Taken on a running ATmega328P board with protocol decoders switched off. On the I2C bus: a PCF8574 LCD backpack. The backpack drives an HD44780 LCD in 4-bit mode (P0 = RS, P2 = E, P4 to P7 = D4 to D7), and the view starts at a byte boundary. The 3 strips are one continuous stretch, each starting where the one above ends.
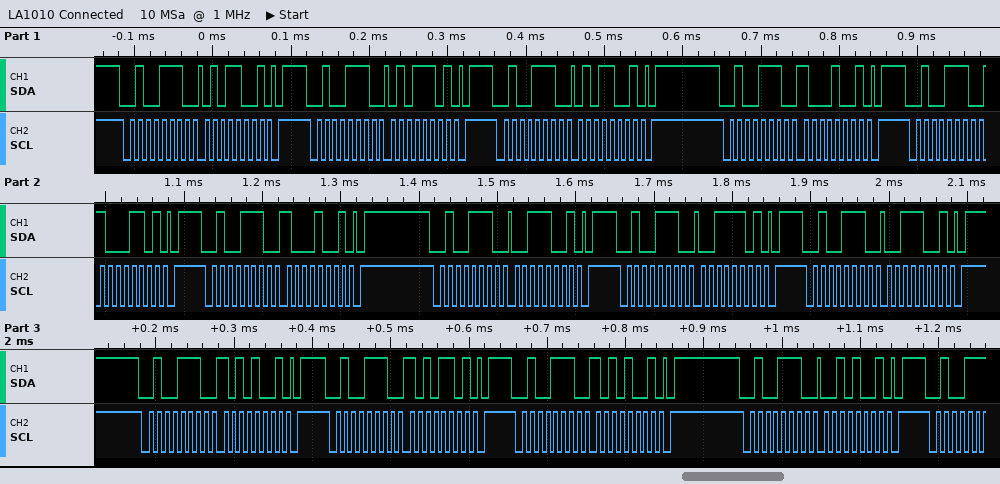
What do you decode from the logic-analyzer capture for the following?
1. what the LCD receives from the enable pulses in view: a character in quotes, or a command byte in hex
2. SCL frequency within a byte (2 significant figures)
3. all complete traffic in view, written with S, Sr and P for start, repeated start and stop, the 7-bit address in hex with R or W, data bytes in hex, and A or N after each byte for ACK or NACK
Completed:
'X' ':'
100 kHz
S 27W A 59 A P S 27W A 5D A P S 27W A 59 A P S 27W A 89 A P S 27W A 8D A P S 27W A 89 A P S 27W A 39 A P S 27W A 3D A P S 27W A 39 A P S 27W A A9 A P S 27W A AD A P S 27W A A9 A P S 27W A 29 A P
